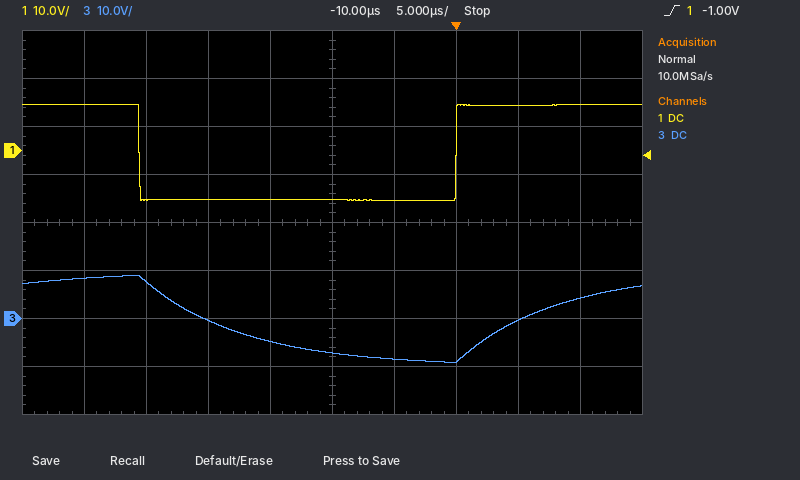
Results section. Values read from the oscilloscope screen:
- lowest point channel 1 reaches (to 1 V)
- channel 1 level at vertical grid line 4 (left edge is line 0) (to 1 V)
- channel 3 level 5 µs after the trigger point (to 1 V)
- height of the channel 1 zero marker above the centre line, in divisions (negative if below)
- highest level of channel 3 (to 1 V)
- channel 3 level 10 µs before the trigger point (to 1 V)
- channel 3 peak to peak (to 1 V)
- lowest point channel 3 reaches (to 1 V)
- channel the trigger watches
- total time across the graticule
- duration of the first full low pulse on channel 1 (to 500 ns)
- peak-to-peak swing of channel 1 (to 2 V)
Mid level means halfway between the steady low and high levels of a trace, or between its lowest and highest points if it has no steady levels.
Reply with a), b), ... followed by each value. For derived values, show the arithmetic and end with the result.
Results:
a) -10 V
b) -10 V
c) 0 V
d) +1.5 div
e) 9 V
f) -7 V
g) 9 V − (-9 V) = 18 V
h) -9 V
i) channel 1
j) 50 µs
k) 25.5 µs
l) 20 V
